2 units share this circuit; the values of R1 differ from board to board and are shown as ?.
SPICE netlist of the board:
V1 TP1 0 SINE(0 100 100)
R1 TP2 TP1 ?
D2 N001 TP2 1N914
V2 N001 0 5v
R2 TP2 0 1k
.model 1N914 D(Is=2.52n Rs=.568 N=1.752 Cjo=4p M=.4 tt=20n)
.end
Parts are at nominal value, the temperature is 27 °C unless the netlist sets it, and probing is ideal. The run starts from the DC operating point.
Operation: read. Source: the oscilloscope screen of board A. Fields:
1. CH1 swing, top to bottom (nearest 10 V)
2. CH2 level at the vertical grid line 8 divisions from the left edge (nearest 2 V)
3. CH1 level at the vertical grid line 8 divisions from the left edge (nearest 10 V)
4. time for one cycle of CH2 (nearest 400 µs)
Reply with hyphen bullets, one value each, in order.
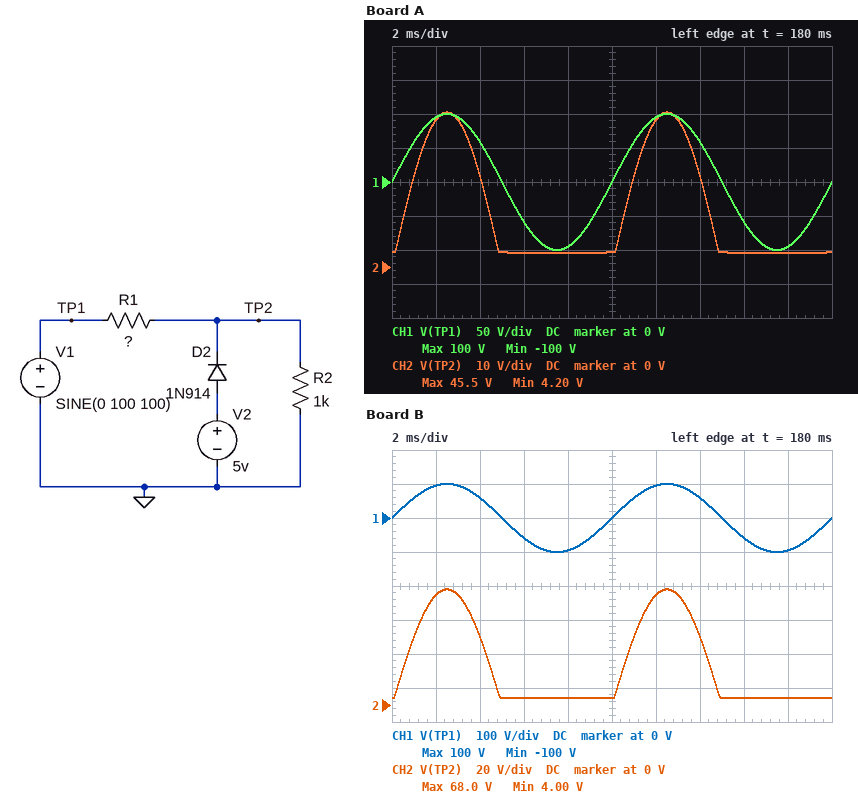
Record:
- 200 V
- 4 V
- -60 V
- 10.0 ms
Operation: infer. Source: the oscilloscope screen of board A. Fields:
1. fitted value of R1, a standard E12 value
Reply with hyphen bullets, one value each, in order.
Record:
- 1.2 kΩ
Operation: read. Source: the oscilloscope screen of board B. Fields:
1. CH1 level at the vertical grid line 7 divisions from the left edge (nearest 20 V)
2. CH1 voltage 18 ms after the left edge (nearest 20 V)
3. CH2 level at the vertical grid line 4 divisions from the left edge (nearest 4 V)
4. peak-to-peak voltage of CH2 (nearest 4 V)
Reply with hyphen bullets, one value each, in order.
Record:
- 60 V
- -100 V
- 4 V
- 64 V
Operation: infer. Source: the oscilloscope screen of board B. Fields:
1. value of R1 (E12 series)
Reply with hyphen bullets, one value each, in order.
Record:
- 470 Ω
